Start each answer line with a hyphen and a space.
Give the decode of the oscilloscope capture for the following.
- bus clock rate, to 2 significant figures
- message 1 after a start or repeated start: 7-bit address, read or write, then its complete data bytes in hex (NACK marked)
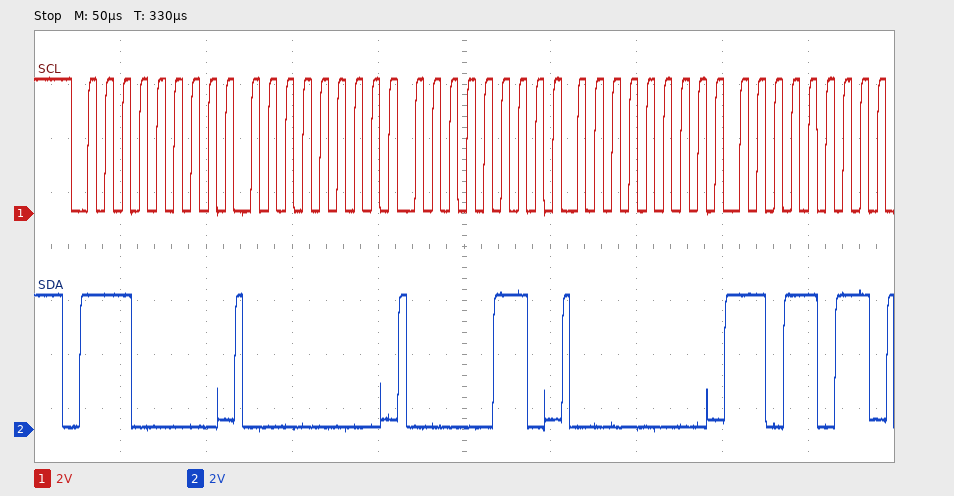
- 100 kHz
- 0x70 write: 00 06 00 DB
